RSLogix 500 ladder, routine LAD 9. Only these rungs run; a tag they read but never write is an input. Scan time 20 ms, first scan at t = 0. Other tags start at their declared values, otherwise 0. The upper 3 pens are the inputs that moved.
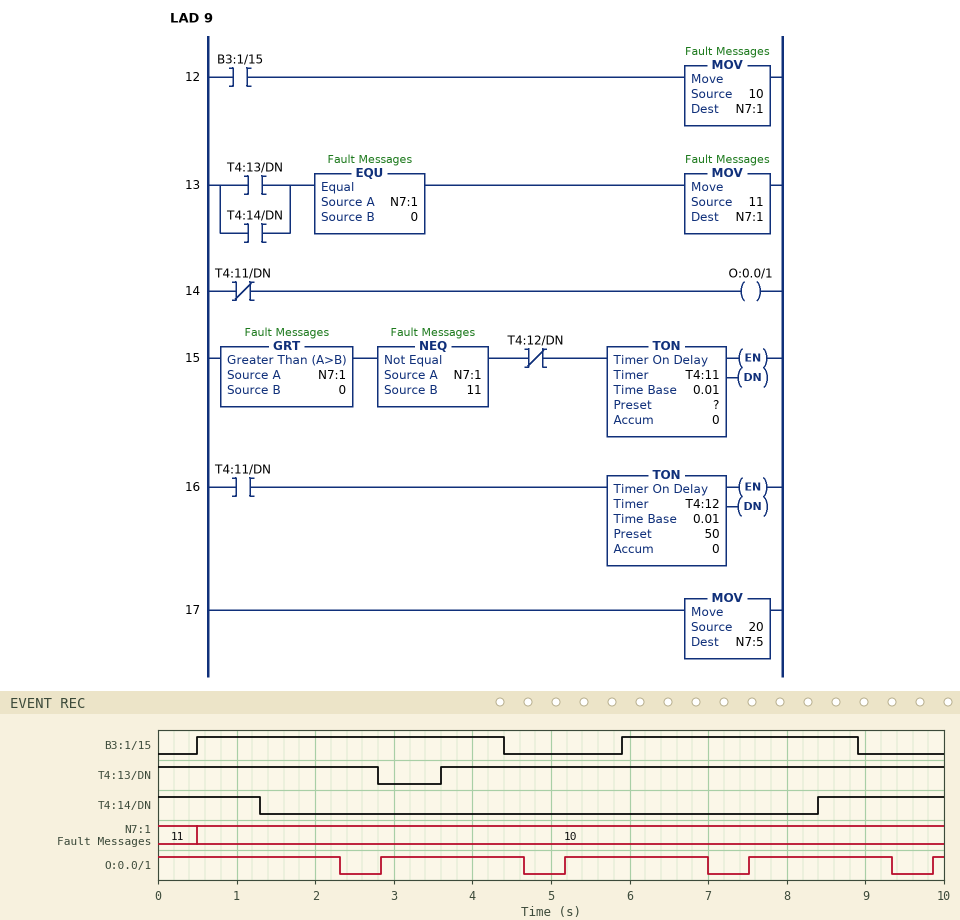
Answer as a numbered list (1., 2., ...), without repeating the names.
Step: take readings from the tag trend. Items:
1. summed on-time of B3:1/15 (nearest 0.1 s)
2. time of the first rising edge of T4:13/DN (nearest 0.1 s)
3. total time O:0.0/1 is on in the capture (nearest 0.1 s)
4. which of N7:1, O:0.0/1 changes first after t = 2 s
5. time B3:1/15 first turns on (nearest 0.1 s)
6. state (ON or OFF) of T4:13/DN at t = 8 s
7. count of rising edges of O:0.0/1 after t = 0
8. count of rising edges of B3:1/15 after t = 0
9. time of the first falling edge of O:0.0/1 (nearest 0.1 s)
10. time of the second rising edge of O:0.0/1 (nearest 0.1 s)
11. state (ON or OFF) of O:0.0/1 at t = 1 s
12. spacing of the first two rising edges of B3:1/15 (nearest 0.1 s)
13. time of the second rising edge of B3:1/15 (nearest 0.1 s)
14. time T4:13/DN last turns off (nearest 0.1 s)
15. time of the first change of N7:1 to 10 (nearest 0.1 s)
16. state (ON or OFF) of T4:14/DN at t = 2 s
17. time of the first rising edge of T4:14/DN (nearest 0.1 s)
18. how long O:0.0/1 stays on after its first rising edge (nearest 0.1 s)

1. 6.9 s
2. 3.6 s
3. 7.9 s
4. O:0.0/1
5. 0.5 s
6. ON
7. 4
8. 2
9. 2.3 s
10. 5.2 s
11. ON
12. 5.4 s
13. 5.9 s
14. 2.8 s
15. 0.5 s
16. OFF
17. 8.4 s
18. 1.8 s
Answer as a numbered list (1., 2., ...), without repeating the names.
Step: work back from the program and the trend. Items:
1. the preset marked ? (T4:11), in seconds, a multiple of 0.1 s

1. 1.8 s
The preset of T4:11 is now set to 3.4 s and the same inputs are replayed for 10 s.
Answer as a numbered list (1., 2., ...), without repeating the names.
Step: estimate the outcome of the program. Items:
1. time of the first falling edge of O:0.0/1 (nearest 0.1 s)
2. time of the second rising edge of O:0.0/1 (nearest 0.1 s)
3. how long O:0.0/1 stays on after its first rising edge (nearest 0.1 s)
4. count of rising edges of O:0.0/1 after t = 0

1. 3.9 s
2. 8.4 s
3. 3.4 s
4. 2
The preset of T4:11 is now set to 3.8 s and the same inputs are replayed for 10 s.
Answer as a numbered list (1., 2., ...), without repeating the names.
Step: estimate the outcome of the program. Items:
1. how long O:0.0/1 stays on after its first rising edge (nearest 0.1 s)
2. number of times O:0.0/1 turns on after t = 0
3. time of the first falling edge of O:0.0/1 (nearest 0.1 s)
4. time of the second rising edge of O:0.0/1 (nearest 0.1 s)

1. 3.8 s
2. 2
3. 4.3 s
4. 9.2 s
